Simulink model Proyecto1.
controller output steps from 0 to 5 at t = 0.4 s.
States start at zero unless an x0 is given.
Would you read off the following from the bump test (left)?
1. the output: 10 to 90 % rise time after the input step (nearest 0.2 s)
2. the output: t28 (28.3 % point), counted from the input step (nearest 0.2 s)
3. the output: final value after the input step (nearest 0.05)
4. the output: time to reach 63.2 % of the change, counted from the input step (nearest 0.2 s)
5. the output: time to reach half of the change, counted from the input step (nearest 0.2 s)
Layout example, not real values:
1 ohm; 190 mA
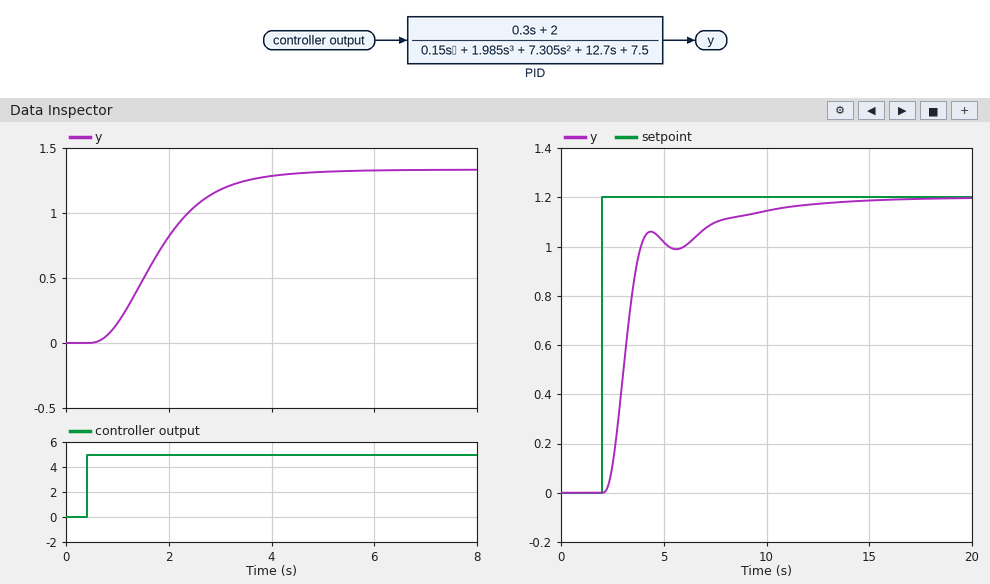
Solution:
2.2 s; 1.0 s; 1.35; 1.6 s; 1.4 s
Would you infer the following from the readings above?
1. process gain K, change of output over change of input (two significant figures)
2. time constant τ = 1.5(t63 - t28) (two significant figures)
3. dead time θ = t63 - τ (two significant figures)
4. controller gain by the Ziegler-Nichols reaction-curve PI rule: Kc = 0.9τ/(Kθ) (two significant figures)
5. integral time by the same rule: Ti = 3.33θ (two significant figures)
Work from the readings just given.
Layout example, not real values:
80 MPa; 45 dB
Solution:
0.27; 0.90 s; 0.70 s; 4.3; 2.3 s
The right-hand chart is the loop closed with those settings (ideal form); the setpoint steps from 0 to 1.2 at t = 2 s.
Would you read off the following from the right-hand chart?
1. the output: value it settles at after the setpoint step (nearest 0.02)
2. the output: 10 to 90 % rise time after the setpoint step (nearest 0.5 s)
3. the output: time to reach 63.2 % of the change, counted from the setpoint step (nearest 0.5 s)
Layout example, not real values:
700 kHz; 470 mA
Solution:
1.20; 4.5 s; 1.5 s
